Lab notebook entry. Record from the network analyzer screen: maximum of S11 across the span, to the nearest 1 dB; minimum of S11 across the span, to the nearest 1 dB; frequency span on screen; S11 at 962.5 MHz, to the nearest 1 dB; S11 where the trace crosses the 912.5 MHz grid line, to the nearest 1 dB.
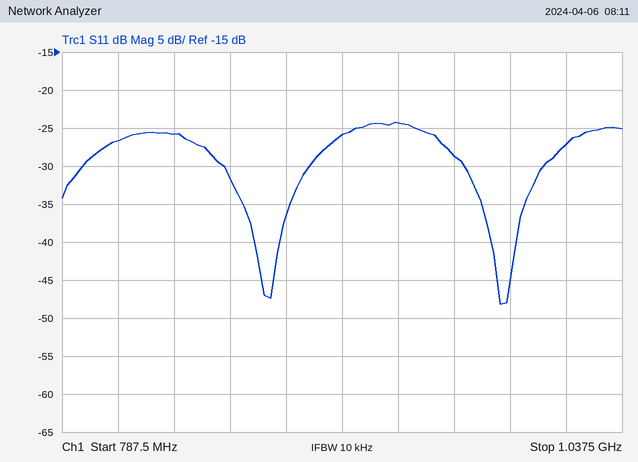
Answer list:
-24 dB
-48 dB
250 MHz
-29 dB
-26 dB
